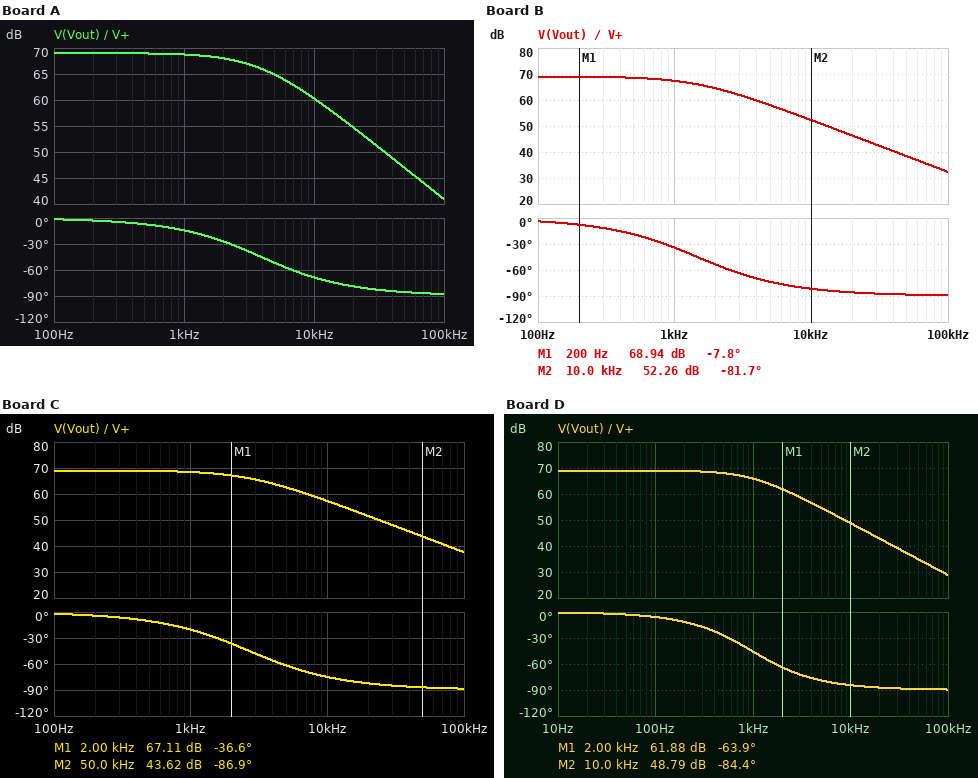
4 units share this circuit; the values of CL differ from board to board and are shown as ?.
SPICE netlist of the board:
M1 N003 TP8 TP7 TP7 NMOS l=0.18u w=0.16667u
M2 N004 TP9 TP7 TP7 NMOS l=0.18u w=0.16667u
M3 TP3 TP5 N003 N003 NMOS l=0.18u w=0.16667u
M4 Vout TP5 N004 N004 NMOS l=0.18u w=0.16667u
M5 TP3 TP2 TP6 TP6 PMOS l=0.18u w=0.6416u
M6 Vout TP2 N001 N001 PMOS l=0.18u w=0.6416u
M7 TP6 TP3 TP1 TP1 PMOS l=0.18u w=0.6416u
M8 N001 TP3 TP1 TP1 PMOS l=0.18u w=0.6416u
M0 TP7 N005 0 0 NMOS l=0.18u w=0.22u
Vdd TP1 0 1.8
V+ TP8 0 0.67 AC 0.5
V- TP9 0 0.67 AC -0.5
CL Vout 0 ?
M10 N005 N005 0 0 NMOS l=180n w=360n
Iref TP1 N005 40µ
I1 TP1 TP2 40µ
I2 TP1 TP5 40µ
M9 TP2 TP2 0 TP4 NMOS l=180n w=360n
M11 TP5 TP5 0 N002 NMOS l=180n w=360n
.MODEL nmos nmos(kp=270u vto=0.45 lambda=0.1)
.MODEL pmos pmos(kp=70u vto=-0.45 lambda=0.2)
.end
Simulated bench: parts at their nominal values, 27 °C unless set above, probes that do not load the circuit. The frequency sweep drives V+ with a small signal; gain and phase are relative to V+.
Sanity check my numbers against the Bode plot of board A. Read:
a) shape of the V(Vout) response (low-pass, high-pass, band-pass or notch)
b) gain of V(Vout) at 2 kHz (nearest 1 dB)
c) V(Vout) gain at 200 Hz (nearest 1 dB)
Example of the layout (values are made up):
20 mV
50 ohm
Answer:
low-pass
68 dB
69 dB
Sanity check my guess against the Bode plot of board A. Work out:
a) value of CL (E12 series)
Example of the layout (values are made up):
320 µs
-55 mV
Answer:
820 fF
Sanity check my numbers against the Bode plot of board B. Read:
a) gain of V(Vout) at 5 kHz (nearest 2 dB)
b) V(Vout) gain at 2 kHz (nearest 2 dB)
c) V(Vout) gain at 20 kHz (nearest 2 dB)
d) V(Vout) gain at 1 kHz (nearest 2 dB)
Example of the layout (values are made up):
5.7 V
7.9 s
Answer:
58 dB
64 dB
46 dB
68 dB
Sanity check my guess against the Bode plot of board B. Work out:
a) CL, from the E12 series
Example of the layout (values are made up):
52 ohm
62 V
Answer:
2.2 pF
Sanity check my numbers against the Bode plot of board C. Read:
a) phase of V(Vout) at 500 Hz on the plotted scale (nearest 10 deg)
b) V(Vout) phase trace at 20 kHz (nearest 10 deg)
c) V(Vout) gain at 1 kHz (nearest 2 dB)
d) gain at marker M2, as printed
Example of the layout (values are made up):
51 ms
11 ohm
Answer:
-10 deg
-80 deg
68 dB
43.62 dB
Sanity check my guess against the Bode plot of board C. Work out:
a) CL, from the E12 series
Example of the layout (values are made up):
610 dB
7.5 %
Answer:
1.2 pF
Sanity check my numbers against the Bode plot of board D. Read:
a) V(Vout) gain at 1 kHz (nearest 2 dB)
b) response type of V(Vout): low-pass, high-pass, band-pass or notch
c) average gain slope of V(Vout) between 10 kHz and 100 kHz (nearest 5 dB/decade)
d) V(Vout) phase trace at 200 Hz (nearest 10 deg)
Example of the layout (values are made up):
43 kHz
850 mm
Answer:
66 dB
low-pass
-20 dB/decade
-10 deg
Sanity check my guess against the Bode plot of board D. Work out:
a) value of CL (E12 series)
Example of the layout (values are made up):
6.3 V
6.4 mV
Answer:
3.3 pF
